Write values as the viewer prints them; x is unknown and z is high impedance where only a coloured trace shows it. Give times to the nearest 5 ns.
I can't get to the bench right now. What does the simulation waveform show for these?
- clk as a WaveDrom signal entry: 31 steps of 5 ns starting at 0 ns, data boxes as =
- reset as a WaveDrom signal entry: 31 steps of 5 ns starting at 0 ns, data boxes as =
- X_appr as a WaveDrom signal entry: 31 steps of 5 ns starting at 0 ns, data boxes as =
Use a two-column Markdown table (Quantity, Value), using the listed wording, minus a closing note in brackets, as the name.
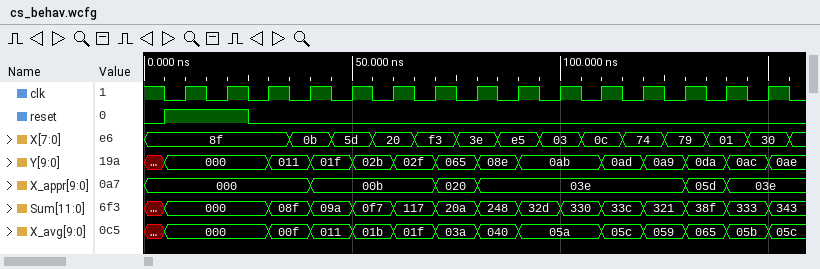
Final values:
| Quantity | Value |
|---|---|
| clk as a WaveDrom signal entry: 31 steps of 5 ns starting at 0 ns, data boxes as = | {name: 'clk', wave: '1010101010101010101010101010101'} |
| reset as a WaveDrom signal entry: 31 steps of 5 ns starting at 0 ns, data boxes as = | {name: 'reset', wave: '01...0.........................'} |
| X_appr as a WaveDrom signal entry: 31 steps of 5 ns starting at 0 ns, data boxes as = | {name: 'X_appr', wave: '=.......=.....=.=.........=.=..', data: '000 00b 020 03e 05d 03e'} |
